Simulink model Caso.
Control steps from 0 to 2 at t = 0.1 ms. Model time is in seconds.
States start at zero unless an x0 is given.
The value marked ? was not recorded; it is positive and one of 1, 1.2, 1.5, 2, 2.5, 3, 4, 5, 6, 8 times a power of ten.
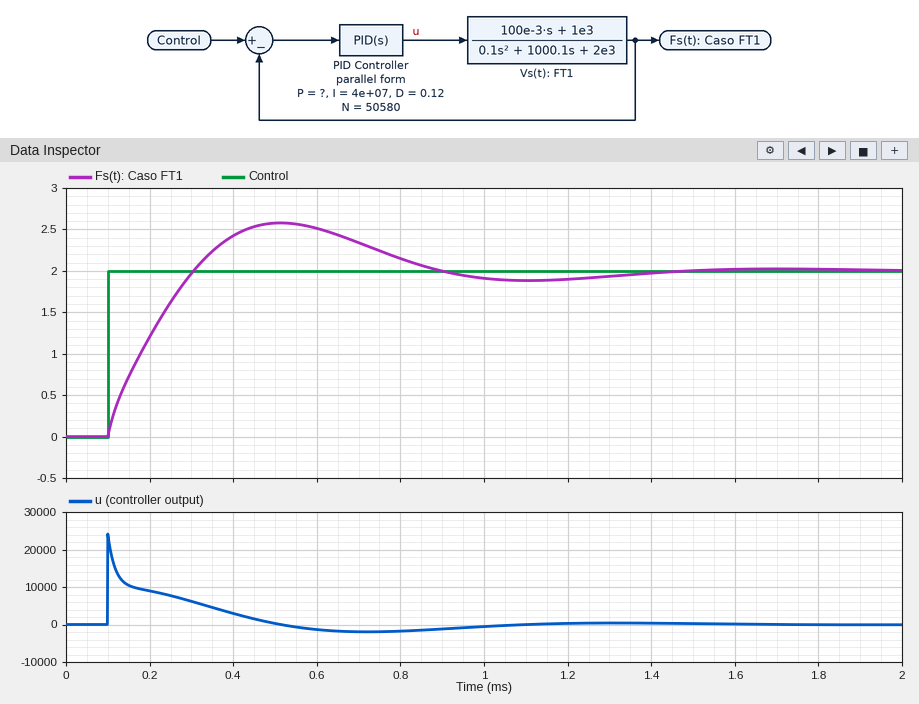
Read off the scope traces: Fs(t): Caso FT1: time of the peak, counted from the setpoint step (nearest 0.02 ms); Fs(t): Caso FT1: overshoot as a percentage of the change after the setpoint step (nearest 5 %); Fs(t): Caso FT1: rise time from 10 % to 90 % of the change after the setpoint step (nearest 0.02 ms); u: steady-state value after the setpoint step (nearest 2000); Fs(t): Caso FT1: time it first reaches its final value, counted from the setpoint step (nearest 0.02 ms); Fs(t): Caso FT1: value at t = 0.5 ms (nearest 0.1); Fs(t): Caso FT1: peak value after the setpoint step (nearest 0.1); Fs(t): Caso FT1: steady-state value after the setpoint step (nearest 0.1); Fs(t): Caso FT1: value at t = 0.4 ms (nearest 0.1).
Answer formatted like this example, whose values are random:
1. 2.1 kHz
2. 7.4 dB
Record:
1. 0.42 ms
2. 30 %
3. 0.16 ms
4. 0
5. 0.20 ms
6. 2.6
7. 2.6
8. 2.0
9. 2.4
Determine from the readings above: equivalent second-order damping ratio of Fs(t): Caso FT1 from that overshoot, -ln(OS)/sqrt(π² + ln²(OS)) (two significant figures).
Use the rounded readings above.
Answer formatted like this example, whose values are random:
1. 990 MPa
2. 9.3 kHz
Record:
1. 0.36
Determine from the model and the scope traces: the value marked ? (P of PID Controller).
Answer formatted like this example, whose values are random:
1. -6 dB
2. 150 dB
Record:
1. 6000
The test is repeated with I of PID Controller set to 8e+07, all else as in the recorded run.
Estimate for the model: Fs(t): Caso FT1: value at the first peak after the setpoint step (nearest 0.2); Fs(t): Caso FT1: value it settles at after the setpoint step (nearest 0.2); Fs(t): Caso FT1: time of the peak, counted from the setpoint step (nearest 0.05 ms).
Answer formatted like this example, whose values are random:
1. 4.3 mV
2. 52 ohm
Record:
1. 2.8
2. 2.0
3. 0.30 ms
